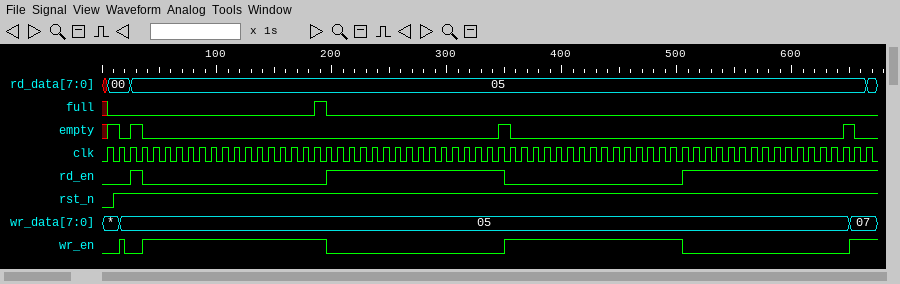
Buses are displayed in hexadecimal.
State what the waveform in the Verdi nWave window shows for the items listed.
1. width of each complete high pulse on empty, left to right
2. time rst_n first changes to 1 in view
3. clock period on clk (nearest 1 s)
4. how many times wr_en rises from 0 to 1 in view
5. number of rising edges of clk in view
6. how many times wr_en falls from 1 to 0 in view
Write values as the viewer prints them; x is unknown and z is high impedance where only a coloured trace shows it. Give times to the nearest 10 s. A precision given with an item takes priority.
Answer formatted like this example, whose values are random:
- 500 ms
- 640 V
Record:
- 10 s, 10 s, 10 s
- 10 s
- 10 s
- 4
- 67
- 3
